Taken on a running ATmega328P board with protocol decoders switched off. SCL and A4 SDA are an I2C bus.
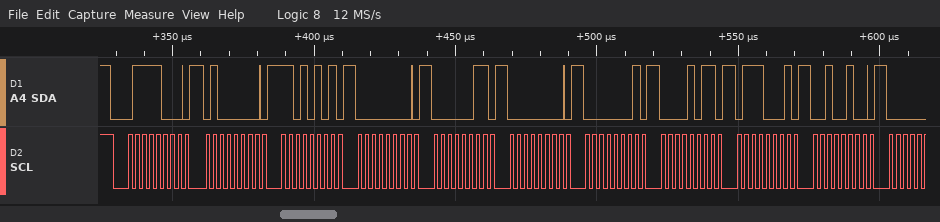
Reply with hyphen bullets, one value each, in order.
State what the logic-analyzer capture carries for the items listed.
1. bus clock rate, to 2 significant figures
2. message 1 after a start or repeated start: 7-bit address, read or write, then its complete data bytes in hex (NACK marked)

- 400 kHz
- 0x3C write: 40 D5 00 03 00 01 0B 71 24
